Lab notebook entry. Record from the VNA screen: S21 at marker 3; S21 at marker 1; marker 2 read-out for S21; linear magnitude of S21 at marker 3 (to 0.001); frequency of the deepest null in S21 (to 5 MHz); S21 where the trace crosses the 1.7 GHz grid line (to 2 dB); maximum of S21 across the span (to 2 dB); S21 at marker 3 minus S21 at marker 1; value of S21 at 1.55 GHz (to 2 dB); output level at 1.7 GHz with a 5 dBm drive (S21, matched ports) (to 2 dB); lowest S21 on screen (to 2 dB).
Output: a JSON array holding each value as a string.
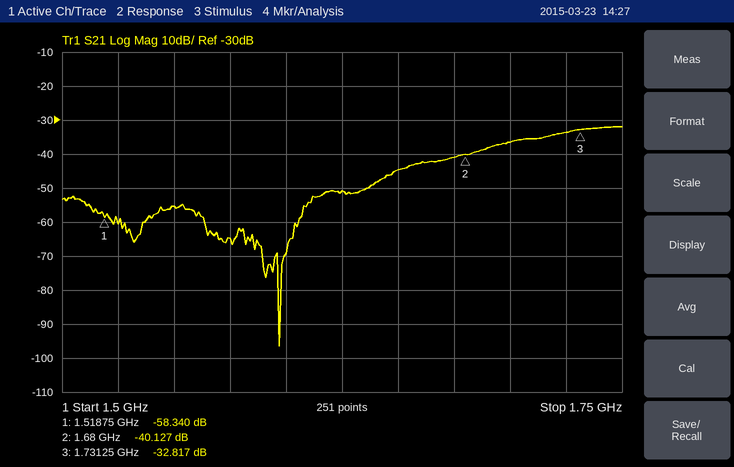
["-32.817 dB", "-58.340 dB", "-40.127 dB", "0.023", "1.595 GHz", "-36 dB", "-32 dB", "25.523 dB", "-56 dB", "-32 dBm", "-96 dB"]
